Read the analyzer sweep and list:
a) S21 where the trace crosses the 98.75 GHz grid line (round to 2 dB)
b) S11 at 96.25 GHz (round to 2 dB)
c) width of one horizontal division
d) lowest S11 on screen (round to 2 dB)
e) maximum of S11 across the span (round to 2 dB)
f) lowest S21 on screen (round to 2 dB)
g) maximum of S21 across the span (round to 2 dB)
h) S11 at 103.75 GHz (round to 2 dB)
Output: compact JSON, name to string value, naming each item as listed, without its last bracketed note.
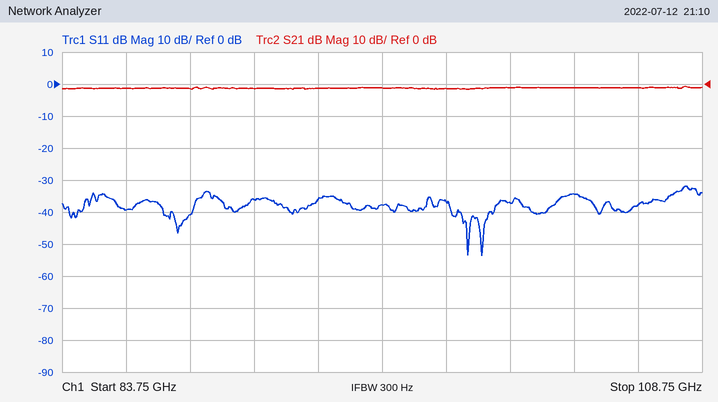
{"S21 where the trace crosses the 98.75 GHz grid line": "-2 dB", "S11 at 96.25 GHz": "-38 dB", "width of one horizontal division": "2.5 GHz", "lowest S11 on screen": "-54 dB", "maximum of S11 across the span": "-32 dB", "lowest S21 on screen": "-2 dB", "maximum of S21 across the span": "0 dB", "S11 at 103.75 GHz": "-34 dB"}
